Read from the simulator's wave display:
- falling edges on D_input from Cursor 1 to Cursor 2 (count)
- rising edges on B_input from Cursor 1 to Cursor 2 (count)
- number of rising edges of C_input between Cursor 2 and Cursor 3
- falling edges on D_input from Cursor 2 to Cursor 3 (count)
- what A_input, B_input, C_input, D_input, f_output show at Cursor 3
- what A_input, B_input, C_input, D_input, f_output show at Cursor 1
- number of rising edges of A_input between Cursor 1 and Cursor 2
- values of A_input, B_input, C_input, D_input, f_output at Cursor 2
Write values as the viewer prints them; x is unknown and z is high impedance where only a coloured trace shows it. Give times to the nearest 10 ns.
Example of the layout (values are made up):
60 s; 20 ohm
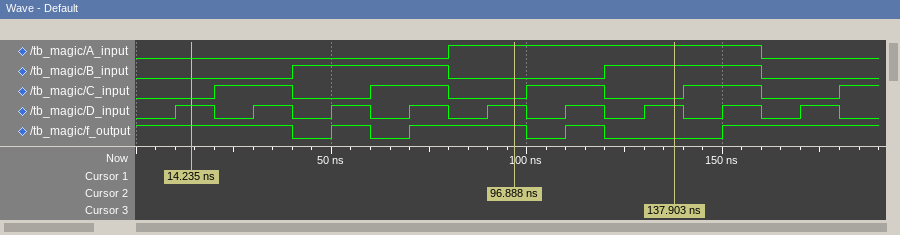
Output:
4; 1; 1; 2; A_input=1, B_input=1, C_input=0, D_input=1, f_output=0; A_input=0, B_input=0, C_input=0, D_input=1, f_output=1; 1; A_input=1, B_input=0, C_input=0, D_input=1, f_output=1
